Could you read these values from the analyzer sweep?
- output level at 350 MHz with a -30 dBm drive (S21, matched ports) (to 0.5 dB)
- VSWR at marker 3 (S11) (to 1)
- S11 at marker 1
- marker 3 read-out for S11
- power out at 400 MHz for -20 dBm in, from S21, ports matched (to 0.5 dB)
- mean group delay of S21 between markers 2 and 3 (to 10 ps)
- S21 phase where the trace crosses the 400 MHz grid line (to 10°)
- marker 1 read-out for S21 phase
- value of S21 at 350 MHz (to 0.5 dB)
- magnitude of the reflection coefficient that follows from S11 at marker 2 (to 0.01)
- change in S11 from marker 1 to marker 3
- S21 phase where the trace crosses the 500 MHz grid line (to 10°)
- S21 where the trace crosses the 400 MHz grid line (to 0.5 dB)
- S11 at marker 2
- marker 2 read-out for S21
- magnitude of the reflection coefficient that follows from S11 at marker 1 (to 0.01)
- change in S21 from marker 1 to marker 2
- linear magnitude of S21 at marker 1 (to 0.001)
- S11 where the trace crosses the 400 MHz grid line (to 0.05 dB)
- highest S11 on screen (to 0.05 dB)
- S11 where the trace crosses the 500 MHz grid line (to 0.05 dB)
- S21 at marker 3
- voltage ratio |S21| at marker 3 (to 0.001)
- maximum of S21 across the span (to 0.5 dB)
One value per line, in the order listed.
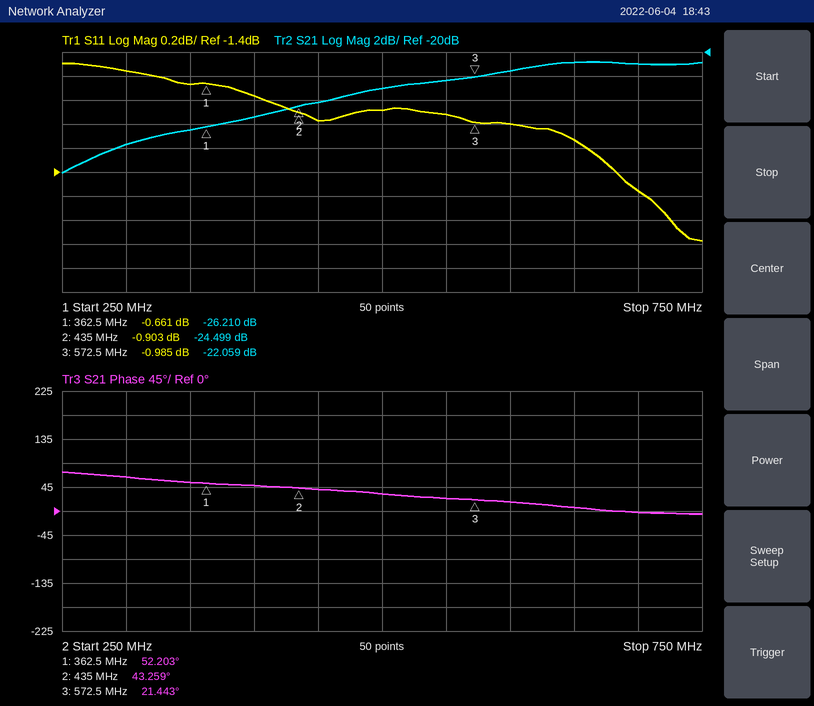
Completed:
-56.5 dBm
18
-0.661 dB
-0.985 dB
-45.5 dBm
440 ps
50°
52.203°
-26.5 dB
0.90
-0.324 dB
30°
-25.5 dB
-0.903 dB
-24.499 dB
0.93
1.711 dB
0.049
-0.75 dB
-0.50 dB
-0.90 dB
-22.059 dB
0.079
-21.0 dB
